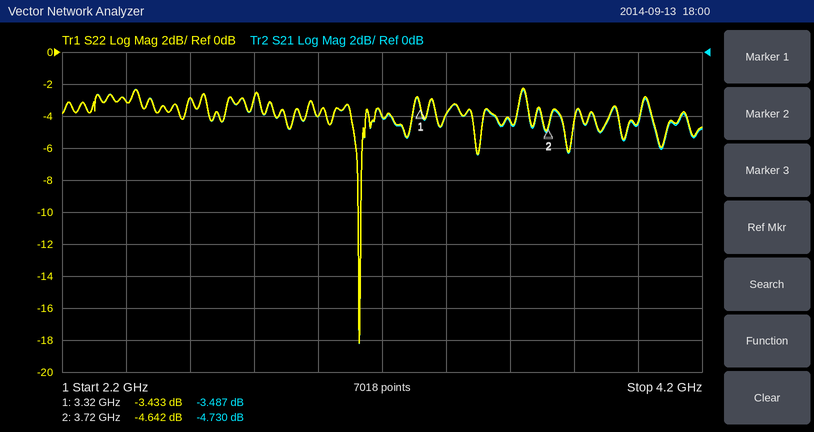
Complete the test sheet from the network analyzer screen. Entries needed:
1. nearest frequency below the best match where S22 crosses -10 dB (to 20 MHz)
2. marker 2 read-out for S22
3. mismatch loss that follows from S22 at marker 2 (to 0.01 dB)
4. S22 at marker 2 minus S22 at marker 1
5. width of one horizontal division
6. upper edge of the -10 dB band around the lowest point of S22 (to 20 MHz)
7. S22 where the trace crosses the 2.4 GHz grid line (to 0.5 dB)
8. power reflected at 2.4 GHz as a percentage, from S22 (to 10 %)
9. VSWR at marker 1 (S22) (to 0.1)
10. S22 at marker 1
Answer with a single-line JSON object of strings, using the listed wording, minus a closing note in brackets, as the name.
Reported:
{"nearest frequency below the best match where S22 crosses -10 dB": "3.12 GHz", "marker 2 read-out for S22": "-4.642 dB", "mismatch loss that follows from S22 at marker 2": "1.83 dB", "S22 at marker 2 minus S22 at marker 1": "-1.209 dB", "width of one horizontal division": "200 MHz", "upper edge of the -10 dB band around the lowest point of S22": "3.14 GHz", "S22 where the trace crosses the 2.4 GHz grid line": "-3.0 dB", "power reflected at 2.4 GHz as a percentage, from S22": "50 %", "VSWR at marker 1 (S22)": "5.1", "S22 at marker 1": "-3.433 dB"}
